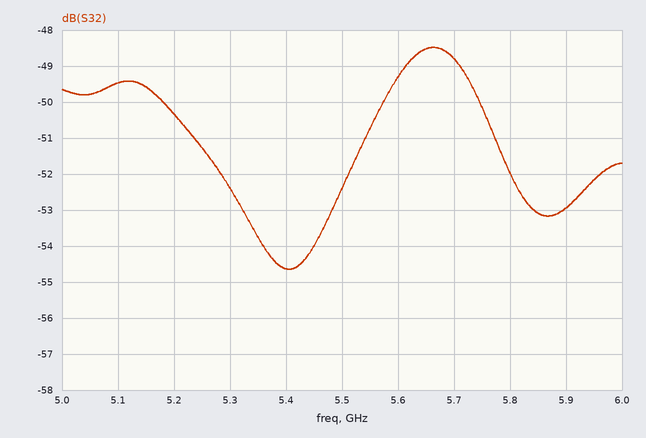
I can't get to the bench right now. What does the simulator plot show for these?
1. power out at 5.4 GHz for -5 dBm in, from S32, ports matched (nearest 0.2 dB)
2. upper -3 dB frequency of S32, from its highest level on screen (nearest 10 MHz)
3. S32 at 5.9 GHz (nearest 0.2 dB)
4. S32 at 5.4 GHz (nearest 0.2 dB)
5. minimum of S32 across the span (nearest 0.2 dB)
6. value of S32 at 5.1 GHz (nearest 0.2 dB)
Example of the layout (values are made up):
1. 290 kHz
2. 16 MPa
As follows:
1. -59.6 dBm
2. 5.79 GHz
3. -53.0 dB
4. -54.6 dB
5. -54.6 dB
6. -49.4 dB
